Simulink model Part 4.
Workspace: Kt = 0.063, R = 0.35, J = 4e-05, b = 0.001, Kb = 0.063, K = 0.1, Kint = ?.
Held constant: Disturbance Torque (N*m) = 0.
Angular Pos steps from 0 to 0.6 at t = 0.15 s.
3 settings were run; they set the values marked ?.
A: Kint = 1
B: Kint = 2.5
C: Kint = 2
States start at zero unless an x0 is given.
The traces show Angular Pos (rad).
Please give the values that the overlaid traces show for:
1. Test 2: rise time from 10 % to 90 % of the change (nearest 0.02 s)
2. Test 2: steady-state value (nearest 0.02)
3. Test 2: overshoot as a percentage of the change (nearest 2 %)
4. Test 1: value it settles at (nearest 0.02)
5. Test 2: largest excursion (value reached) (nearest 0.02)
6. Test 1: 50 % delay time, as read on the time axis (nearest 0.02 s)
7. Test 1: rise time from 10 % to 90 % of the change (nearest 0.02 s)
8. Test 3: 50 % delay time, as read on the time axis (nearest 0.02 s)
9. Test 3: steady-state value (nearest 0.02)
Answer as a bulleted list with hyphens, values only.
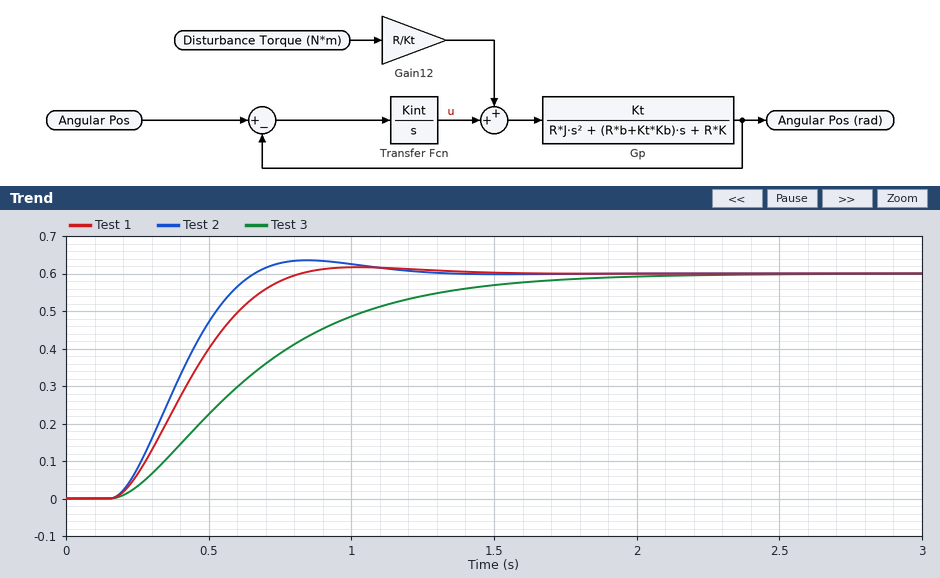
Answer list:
- 0.34 s
- 0.60
- 6 %
- 0.60
- 0.64
- 0.42 s
- 0.42 s
- 0.60 s
- 0.60
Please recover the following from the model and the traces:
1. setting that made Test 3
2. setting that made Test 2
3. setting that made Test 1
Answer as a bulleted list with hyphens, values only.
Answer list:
- A
- B
- C
